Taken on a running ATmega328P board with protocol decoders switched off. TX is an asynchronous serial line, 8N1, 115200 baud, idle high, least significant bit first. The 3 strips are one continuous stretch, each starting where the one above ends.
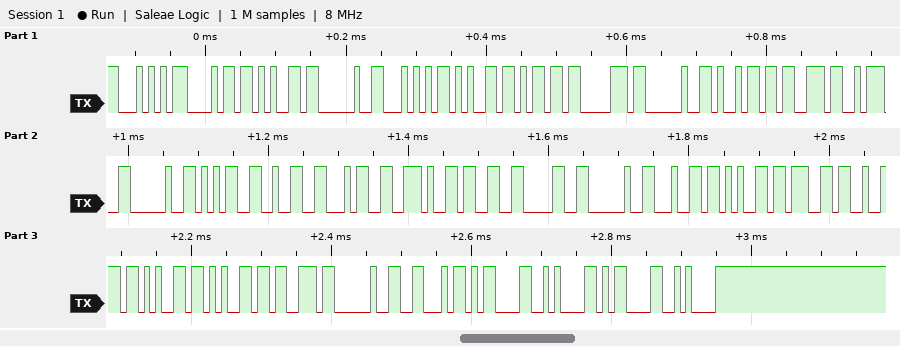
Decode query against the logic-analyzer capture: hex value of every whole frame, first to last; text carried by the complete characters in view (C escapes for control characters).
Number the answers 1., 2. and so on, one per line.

1. 54 68 65 20 54 65 6D 70 20 69 73 3A 20 35 32 34 2E 33 30 20 64 65 67 72 65 65 73 20 46 0D 0A 0D 0A
2. "The Temp is: 524.30 degrees F\r\n\r\n"
